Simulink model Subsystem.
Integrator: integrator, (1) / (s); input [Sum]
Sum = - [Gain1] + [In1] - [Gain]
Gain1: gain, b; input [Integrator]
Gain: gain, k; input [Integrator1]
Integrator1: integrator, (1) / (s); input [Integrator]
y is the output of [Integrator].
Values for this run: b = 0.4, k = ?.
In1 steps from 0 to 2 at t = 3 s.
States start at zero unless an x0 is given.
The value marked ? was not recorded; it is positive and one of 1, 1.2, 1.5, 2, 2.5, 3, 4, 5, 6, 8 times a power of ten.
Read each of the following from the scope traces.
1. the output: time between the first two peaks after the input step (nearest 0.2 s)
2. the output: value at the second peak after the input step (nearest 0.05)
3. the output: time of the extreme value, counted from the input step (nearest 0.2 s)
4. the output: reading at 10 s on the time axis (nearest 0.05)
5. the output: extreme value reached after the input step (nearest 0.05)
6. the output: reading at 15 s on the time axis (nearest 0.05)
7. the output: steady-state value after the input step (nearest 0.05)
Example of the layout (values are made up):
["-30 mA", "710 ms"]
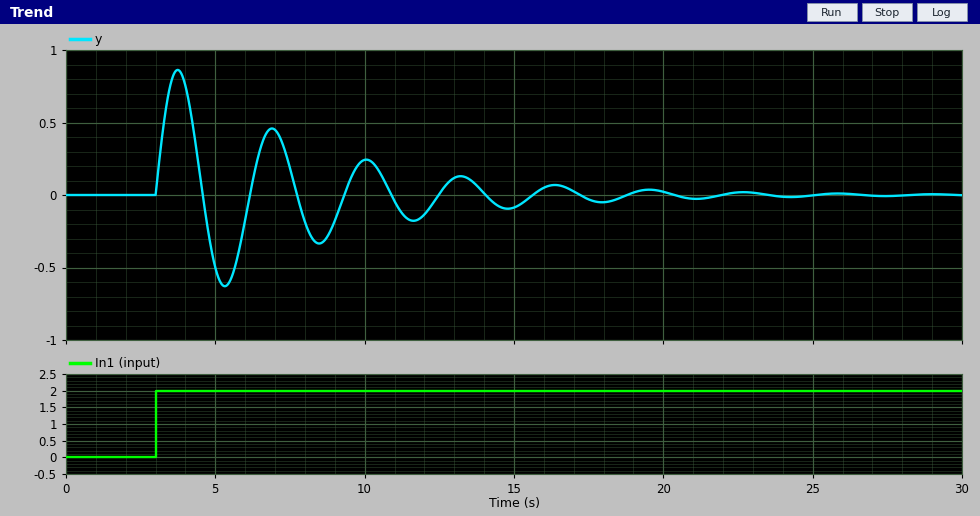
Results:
["3.2 s", "0.45", "0.8 s", "0.25", "0.85", "-0.10", "0.00"]
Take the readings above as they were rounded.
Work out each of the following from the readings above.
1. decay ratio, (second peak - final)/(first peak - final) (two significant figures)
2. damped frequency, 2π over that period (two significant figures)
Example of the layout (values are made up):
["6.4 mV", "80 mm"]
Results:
["0.53", "2.0 rad/s"]
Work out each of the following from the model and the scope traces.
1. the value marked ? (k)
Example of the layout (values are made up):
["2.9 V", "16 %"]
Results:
["4"]
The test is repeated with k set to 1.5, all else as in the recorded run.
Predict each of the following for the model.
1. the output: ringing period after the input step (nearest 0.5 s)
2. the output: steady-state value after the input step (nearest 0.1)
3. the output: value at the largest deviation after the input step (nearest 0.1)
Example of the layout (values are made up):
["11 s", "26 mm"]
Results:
["5.0 s", "0.0", "1.3"]
